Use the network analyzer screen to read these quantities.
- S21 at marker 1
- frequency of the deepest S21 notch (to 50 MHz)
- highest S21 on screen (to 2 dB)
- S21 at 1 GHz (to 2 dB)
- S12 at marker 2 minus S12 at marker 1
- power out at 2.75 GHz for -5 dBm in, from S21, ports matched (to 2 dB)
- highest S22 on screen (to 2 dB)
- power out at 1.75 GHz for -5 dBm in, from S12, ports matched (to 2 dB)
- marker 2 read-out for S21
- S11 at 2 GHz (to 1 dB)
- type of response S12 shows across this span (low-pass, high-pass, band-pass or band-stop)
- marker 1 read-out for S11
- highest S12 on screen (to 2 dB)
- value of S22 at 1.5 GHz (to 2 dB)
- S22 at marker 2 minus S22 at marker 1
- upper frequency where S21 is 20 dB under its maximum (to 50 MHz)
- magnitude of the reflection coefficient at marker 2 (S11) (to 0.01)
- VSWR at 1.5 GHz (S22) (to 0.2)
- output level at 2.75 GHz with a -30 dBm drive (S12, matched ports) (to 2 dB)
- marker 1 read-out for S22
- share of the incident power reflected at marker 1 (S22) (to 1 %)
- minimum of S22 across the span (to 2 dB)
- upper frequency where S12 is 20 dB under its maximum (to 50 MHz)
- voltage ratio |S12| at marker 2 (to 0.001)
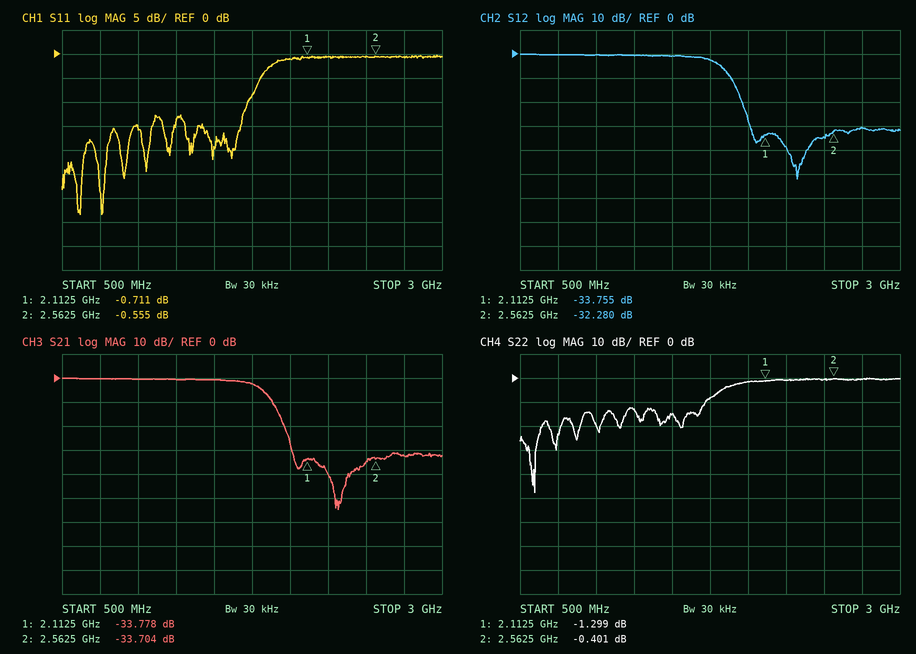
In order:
-33.778 dB
2.30 GHz
0 dB
0 dB
1.475 dB
-38 dBm
0 dB
-8 dBm
-33.704 dB
-1 dB
low-pass
-0.711 dB
0 dB
-16 dB
0.898 dB
1.95 GHz
0.94
1.4
-60 dBm
-1.299 dB
74 %
-48 dB
1.95 GHz
0.024
